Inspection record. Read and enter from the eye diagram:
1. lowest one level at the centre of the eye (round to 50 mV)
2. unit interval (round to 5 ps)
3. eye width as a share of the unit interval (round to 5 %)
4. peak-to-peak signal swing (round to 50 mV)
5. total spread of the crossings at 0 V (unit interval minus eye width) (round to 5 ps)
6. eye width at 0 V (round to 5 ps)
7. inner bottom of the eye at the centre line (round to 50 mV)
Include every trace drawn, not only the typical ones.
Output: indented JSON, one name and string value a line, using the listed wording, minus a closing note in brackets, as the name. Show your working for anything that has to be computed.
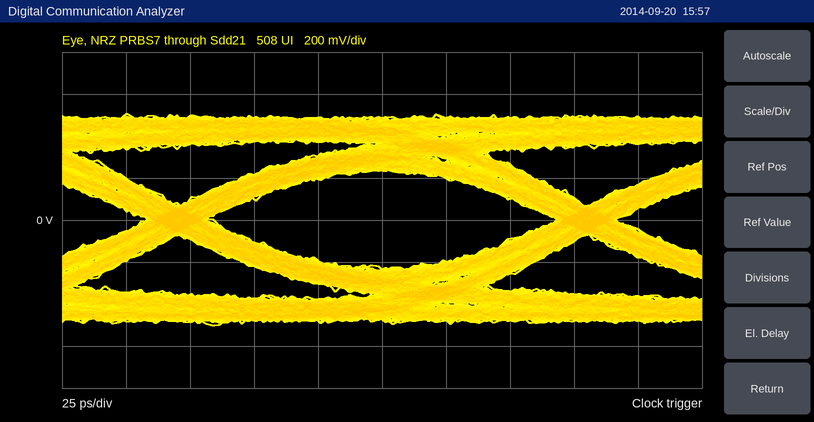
{
  "lowest one level at the centre of the eye": "250 mV",
  "unit interval": "160 ps",
  "eye width as a share of the unit interval": "135 ps / 160 ps ≈ 84.4 %, so 85 % to the nearest 5 %",
  "peak-to-peak signal swing": "1.00 V",
  "total spread of the crossings at 0 V (unit interval minus eye width)": "25 ps",
  "eye width at 0 V": "135 ps",
  "inner bottom of the eye at the centre line": "-250 mV"
}
